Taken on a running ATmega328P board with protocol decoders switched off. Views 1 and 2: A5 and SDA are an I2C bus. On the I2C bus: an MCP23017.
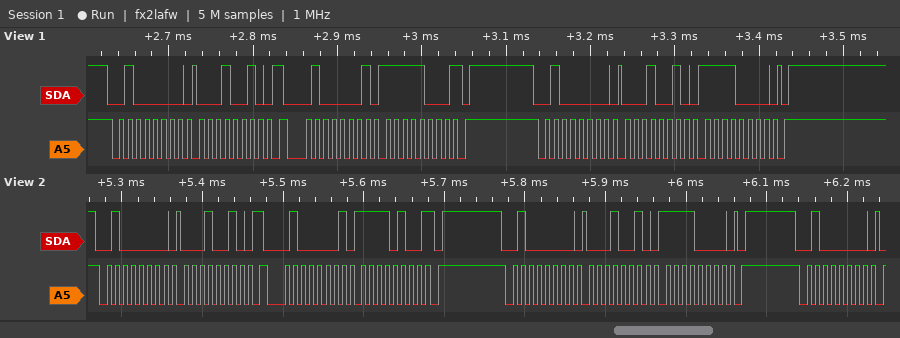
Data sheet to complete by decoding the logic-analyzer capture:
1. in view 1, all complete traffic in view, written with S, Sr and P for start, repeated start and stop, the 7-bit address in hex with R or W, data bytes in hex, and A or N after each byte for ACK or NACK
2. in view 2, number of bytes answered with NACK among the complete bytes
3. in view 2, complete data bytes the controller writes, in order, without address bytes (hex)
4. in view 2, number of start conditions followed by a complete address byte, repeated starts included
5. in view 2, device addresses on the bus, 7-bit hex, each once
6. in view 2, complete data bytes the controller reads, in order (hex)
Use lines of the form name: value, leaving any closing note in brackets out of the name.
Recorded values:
in view 1, all complete traffic in view, written with S, Sr and P for start, repeated start and stop, the 7-bit address in hex with R or W, data bytes in hex, and A or N after each byte for ACK or NACK: S 20W A 12 A Sr 20R A F8 N P S 20W A 12 A F0 A P
in view 2, number of bytes answered with NACK among the complete bytes: 1
in view 2, complete data bytes the controller writes, in order, without address bytes: 12 12 F0
in view 2, number of start conditions followed by a complete address byte, repeated starts included: 4
in view 2, device addresses on the bus, 7-bit hex, each once: 0x20
in view 2, complete data bytes the controller reads, in order: F4
